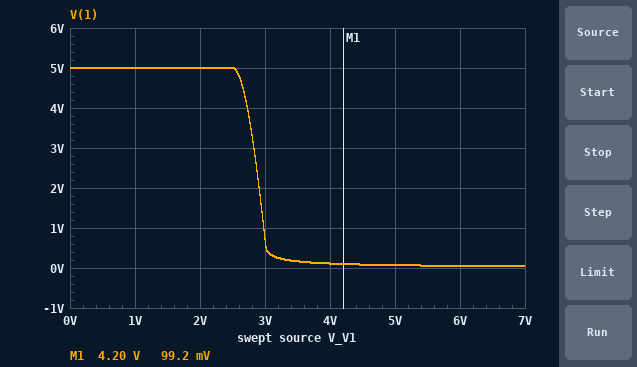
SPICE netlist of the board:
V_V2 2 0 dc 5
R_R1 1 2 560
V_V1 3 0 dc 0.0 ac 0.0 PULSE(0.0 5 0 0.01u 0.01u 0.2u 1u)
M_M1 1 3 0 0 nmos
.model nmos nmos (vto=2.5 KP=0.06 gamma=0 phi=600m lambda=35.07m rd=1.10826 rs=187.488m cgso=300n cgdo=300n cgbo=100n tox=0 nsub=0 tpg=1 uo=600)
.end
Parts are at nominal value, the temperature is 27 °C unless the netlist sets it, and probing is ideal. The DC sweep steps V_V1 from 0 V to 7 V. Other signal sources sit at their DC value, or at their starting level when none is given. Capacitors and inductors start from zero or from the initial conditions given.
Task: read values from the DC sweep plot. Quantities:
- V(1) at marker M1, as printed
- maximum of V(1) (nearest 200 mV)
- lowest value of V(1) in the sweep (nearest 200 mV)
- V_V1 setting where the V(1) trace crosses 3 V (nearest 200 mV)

99.2 mV
5.0 V
0 V
2.8 V
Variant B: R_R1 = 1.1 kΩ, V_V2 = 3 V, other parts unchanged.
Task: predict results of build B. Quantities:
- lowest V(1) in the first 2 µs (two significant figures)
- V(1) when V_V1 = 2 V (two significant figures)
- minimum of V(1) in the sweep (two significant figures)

-720 mV
3.0 V
14 mV
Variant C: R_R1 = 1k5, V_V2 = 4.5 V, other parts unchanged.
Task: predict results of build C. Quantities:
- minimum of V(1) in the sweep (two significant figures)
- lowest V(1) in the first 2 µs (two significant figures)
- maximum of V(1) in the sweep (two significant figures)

15 mV
-720 mV
4.5 V
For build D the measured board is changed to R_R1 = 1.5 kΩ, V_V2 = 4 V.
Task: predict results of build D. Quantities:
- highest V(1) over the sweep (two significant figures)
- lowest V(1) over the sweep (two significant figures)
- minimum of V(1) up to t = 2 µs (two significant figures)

4.0 V
13 mV
-720 mV
